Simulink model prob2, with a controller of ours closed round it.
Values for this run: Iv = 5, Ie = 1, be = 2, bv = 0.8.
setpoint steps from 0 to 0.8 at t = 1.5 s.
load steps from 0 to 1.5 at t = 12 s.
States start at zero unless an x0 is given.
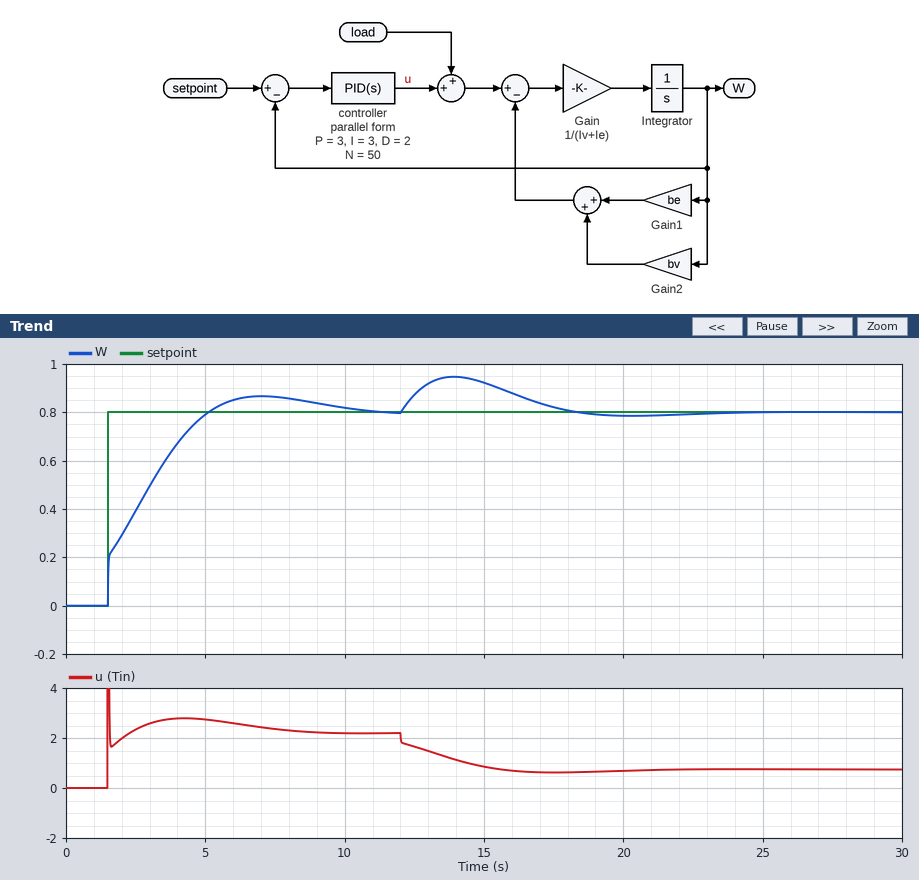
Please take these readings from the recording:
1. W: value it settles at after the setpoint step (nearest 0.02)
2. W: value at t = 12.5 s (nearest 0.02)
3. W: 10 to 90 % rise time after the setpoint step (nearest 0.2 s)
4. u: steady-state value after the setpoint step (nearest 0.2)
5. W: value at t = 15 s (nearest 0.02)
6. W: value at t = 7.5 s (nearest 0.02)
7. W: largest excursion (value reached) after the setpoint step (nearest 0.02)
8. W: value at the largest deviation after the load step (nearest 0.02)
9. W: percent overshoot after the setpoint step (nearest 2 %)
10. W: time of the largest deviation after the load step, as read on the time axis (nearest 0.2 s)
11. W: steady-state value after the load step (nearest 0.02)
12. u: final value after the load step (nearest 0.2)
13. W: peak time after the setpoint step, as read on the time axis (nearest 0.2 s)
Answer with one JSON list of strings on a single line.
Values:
["0.80", "0.88", "2.8 s", "2.2", "0.92", "0.86", "0.86", "0.94", "8 %", "14.0 s", "0.80", "0.8", "7.0 s"]
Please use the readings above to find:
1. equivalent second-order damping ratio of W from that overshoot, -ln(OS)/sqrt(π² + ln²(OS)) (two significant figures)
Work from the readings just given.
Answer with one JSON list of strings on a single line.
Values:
["0.63"]
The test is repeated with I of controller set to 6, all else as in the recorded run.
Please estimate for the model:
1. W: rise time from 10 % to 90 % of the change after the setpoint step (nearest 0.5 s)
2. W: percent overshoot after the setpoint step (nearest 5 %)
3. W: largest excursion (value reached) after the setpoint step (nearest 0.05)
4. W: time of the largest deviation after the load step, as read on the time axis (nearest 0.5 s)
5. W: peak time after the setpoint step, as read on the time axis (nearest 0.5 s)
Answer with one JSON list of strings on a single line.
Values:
["2.0 s", "20 %", "0.95", "13.5 s", "5.0 s"]
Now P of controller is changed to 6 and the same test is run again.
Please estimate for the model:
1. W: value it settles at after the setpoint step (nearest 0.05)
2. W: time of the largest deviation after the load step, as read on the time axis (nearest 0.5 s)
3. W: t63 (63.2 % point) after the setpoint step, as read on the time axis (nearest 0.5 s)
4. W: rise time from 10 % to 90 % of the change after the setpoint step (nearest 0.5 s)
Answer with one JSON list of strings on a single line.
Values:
["0.80", "13.5 s", "2.5 s", "2.5 s"]
